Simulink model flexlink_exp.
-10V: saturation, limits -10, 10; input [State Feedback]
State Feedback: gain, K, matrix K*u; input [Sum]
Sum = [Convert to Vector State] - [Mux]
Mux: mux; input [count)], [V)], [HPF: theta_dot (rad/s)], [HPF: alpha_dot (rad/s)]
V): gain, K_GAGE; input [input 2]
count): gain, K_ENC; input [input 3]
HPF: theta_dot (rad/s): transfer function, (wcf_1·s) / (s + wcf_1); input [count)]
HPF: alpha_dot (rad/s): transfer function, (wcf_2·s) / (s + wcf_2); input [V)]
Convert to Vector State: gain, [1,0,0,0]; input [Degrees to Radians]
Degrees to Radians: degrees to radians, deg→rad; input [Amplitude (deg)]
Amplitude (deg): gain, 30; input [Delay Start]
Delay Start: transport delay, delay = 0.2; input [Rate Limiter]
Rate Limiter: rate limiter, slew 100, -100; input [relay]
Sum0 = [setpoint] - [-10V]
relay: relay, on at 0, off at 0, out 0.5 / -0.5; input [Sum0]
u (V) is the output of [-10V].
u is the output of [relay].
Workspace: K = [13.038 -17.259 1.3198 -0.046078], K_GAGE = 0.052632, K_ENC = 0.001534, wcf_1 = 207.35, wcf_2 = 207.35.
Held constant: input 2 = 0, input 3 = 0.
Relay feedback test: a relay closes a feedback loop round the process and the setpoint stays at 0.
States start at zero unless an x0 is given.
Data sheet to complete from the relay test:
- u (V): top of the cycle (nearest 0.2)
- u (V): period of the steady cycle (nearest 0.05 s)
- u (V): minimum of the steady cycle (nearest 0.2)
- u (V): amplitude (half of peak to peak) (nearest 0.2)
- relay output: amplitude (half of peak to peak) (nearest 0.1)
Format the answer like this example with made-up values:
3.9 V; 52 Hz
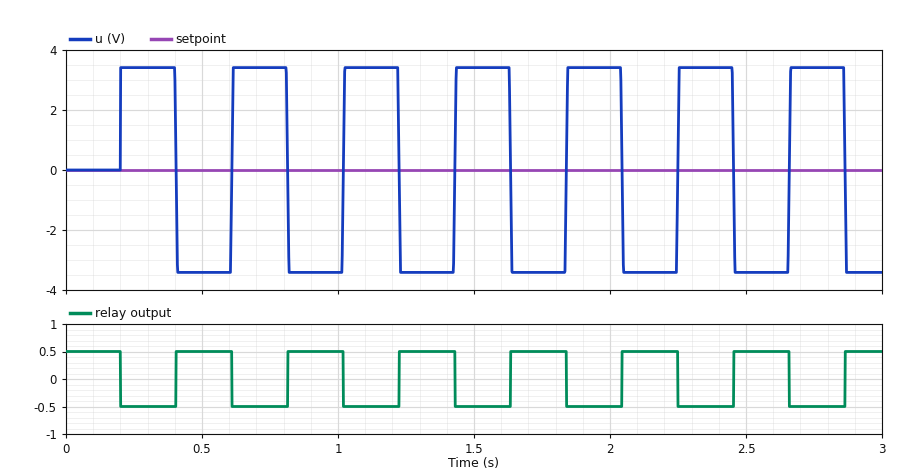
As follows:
3.4; 0.40 s; -3.4; 3.4; 0.5
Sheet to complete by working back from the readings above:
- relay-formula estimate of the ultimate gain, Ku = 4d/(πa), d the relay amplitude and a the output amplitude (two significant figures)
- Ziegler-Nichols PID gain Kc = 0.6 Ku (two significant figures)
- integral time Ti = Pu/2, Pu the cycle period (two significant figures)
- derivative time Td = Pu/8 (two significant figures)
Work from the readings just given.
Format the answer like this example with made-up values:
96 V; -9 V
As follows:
0.19; 0.11; 0.20 s; 0.050 s
